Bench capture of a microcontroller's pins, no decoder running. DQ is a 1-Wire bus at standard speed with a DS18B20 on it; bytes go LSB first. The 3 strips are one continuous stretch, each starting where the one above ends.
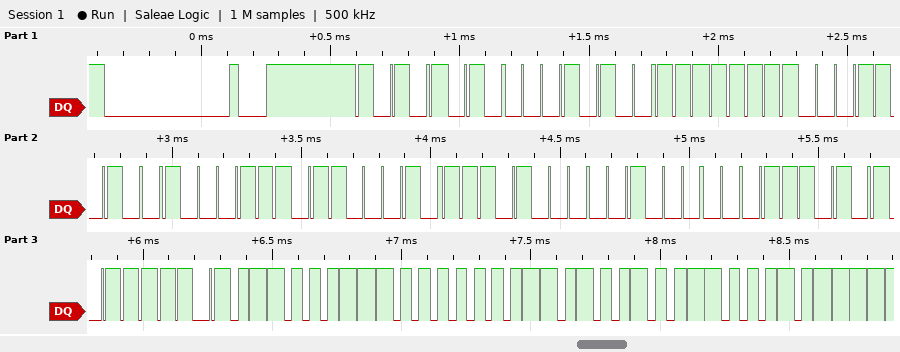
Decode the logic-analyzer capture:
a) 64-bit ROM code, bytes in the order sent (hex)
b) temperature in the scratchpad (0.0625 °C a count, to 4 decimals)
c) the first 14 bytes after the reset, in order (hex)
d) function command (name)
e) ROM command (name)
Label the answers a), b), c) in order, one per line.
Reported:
a) 28 FF 58 E2 46 17 04 AE
b) 28.3750 °C
c) 55 28 FF 58 E2 46 17 04 AE BE C6 01 4B 46
d) Read Scratchpad
e) Match ROM
